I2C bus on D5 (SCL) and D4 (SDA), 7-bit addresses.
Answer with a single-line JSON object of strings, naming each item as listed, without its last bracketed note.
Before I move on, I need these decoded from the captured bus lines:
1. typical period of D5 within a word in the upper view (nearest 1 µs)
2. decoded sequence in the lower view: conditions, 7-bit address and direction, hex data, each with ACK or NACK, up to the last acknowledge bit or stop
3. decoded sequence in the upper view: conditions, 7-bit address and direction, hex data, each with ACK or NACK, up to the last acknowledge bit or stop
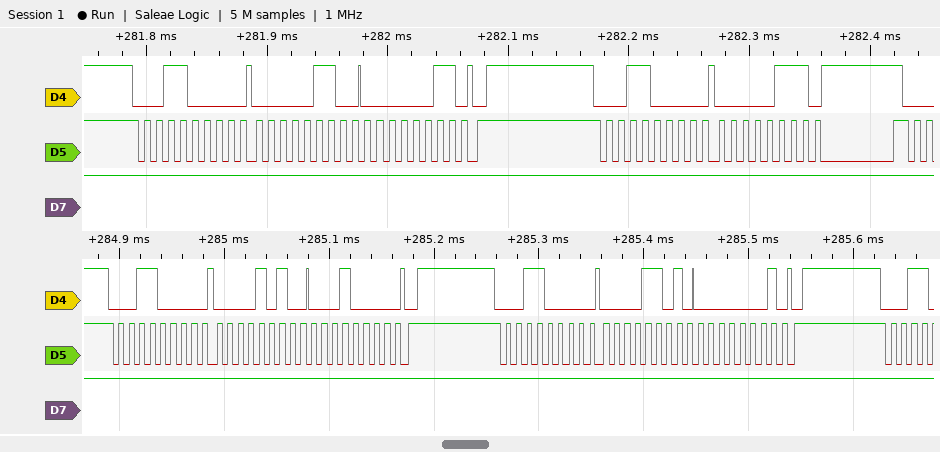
{"typical period of D5 within a word in the upper view": "10 µs", "decoded sequence in the lower view: conditions, 7-bit address and direction, hex data, each with ACK or NACK, up to the last acknowledge bit or stop": "start, address 18 write ACK, 0A ACK, 10 ACK, stop, start, address 18 write ACK, 0D ACK, 01 ACK, stop", "decoded sequence in the upper view: conditions, 7-bit address and direction, hex data, each with ACK or NACK, up to the last acknowledge bit or stop": "start, address 18 write ACK, 06 ACK, 03 ACK, stop, start, address 18 write ACK, 07 ACK"}
